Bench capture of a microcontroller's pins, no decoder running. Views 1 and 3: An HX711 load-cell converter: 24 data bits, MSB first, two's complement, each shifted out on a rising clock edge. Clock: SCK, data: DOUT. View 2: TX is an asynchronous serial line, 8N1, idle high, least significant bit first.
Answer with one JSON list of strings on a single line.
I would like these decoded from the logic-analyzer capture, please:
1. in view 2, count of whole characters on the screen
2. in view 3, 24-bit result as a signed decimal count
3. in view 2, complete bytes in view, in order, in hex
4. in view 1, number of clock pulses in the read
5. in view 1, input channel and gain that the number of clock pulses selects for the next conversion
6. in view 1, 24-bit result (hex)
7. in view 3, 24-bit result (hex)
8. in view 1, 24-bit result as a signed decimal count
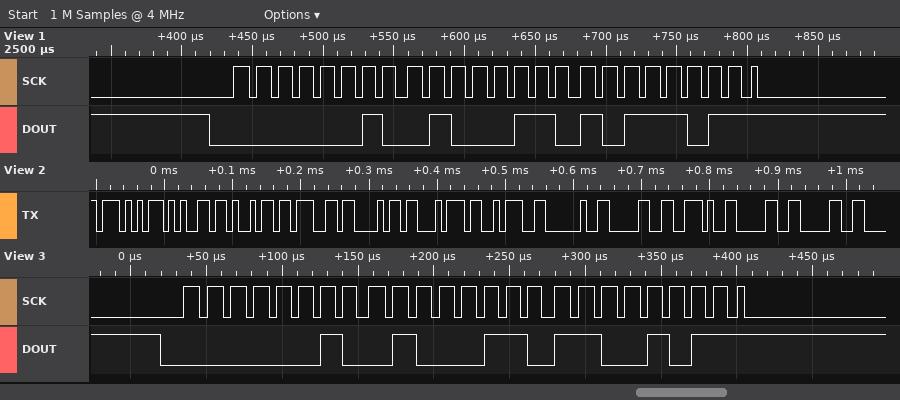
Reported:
["12", "149195", "57 65 69 67 68 74 3A 20 30 2E 30 30", "25", "channel A, gain 128", "0x0246BB", "0x0246CB", "149179"]
